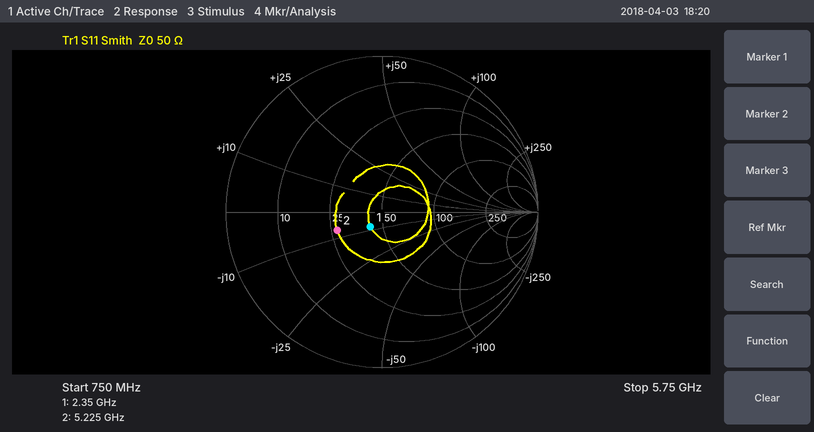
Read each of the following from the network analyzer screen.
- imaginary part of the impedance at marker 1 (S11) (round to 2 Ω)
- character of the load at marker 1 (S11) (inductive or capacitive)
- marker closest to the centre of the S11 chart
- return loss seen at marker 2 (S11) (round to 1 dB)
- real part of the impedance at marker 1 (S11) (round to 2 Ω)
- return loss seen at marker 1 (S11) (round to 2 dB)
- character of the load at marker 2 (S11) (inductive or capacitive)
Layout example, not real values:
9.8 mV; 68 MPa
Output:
-8 Ω; capacitive; marker 1; 10 dB; 42 Ω; 18 dB; capacitive
